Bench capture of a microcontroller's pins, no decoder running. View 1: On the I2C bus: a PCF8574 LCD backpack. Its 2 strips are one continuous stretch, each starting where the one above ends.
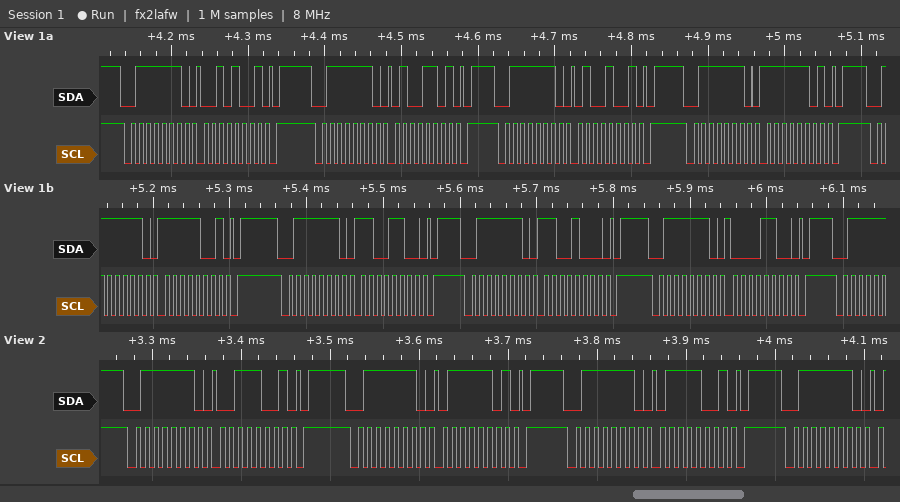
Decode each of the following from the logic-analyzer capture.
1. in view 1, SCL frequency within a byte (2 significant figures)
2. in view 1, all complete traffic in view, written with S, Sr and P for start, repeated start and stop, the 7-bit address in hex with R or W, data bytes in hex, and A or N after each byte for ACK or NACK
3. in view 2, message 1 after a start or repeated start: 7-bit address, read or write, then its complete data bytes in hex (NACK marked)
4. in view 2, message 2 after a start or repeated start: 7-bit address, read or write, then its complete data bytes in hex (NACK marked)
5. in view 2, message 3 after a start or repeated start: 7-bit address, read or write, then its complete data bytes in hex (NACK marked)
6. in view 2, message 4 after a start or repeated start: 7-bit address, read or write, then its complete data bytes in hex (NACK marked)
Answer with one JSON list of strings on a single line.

["100 kHz", "S 3FW A 29 A P S 3FW A 4D A P S 3FW A 49 A P S 3FW A FD A P S 3FW A F9 A P S 3FW A CC A P S 3FW A C8 A P S 3FW A 0C A P", "0x3F write: 39", "0x3F write: 7D", "0x3F write: 79", "0x3F write"]
